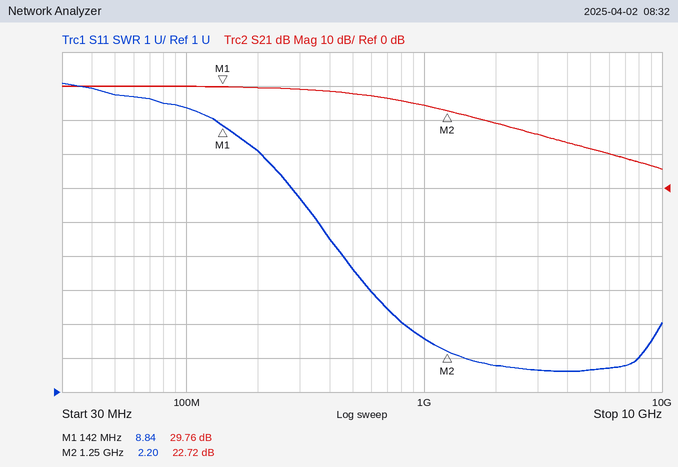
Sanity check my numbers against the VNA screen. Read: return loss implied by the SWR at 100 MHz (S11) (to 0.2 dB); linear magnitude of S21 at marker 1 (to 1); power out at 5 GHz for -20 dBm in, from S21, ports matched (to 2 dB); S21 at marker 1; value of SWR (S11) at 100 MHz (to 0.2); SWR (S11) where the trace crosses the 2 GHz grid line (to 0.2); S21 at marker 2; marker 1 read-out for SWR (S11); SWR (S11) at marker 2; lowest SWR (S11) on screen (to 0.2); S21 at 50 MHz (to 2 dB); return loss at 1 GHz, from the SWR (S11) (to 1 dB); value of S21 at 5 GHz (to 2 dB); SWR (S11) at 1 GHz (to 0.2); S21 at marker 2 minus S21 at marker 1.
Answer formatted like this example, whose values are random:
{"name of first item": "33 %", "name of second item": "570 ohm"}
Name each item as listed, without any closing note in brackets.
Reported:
{"return loss implied by the SWR at 100 MHz (S11)": "1.8 dB", "linear magnitude of S21 at marker 1": "31", "power out at 5 GHz for -20 dBm in, from S21, ports matched": "-8 dBm", "S21 at marker 1": "29.76 dB", "value of SWR (S11) at 100 MHz": "9.4", "SWR (S11) where the trace crosses the 2 GHz grid line": "1.8", "S21 at marker 2": "22.72 dB", "marker 1 read-out for SWR": "8.84", "SWR (S11) at marker 2": "2.20", "lowest SWR (S11) on screen": "1.6", "S21 at 50 MHz": "30 dB", "return loss at 1 GHz, from the SWR (S11)": "7 dB", "value of S21 at 5 GHz": "12 dB", "SWR (S11) at 1 GHz": "2.6", "S21 at marker 2 minus S21 at marker 1": "-7.04 dB"}
